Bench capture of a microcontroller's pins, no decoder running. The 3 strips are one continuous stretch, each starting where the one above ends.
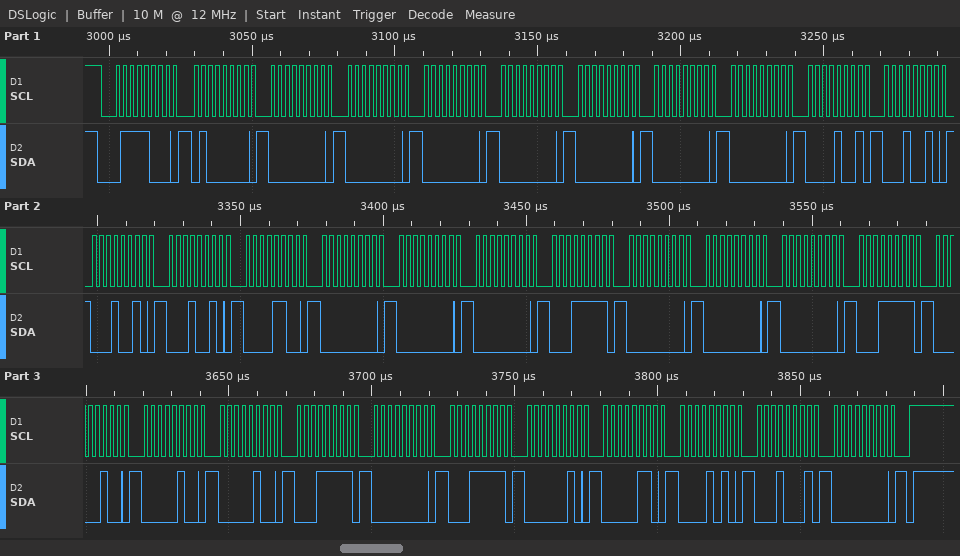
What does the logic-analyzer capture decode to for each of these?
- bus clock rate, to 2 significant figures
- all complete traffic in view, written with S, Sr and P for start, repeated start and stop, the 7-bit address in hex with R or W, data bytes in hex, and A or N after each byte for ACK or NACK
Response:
400 kHz
S 3CW A 40 A 00 A 00 A 00 A 00 A 00 A 00 A 00 A 09 A 12 A 12 A 12 A 0C A 00 A 00 A 00 A 1F A 00 A 00 A 00 A 1F A 04 A 04 A 04 A 1F A 00 A 1F A 02 A 06 A 0A A 11 A 00 A P
